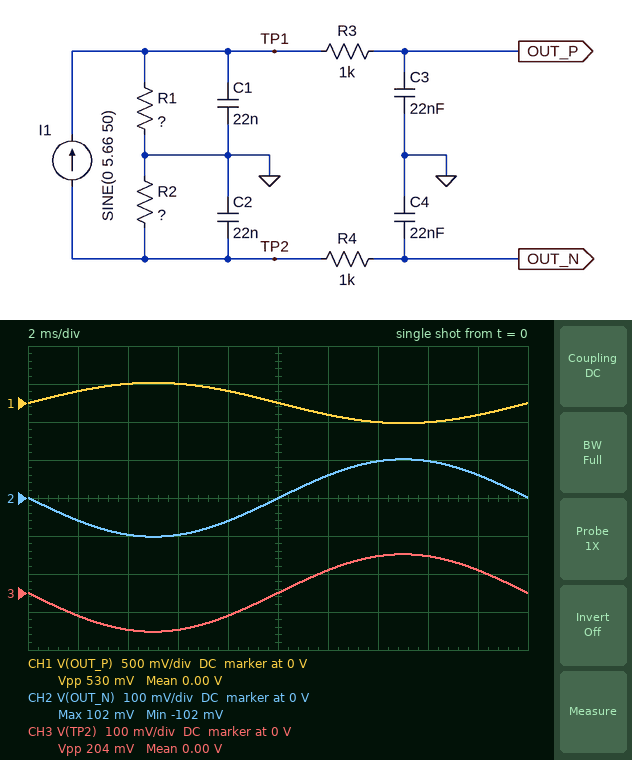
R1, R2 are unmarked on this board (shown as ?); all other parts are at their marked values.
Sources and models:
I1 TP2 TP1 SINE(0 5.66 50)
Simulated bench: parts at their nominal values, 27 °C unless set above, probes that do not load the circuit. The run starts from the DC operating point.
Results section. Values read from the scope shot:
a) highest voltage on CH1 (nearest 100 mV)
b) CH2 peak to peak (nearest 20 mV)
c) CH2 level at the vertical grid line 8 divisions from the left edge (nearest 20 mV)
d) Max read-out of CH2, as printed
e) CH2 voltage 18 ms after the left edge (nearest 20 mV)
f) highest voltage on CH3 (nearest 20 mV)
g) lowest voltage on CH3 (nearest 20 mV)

300 mV
200 mV
100 mV
102 mV
60 mV
100 mV
-100 mV
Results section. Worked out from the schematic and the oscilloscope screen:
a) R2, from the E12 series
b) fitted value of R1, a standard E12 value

0.018 Ω
0.047 Ω
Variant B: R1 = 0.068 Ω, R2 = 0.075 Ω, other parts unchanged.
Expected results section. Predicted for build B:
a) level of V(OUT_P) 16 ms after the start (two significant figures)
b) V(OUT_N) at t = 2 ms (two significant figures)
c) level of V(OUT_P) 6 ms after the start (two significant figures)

-370 mV
-250 mV
370 mV
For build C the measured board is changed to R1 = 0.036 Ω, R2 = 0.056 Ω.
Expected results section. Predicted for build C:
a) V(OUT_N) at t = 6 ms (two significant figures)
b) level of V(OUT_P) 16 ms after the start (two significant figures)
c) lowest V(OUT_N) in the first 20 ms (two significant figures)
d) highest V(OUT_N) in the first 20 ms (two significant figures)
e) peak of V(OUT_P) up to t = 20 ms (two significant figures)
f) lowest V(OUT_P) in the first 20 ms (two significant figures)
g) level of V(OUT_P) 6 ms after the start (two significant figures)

-300 mV
-190 mV
-320 mV
320 mV
200 mV
-200 mV
190 mV
